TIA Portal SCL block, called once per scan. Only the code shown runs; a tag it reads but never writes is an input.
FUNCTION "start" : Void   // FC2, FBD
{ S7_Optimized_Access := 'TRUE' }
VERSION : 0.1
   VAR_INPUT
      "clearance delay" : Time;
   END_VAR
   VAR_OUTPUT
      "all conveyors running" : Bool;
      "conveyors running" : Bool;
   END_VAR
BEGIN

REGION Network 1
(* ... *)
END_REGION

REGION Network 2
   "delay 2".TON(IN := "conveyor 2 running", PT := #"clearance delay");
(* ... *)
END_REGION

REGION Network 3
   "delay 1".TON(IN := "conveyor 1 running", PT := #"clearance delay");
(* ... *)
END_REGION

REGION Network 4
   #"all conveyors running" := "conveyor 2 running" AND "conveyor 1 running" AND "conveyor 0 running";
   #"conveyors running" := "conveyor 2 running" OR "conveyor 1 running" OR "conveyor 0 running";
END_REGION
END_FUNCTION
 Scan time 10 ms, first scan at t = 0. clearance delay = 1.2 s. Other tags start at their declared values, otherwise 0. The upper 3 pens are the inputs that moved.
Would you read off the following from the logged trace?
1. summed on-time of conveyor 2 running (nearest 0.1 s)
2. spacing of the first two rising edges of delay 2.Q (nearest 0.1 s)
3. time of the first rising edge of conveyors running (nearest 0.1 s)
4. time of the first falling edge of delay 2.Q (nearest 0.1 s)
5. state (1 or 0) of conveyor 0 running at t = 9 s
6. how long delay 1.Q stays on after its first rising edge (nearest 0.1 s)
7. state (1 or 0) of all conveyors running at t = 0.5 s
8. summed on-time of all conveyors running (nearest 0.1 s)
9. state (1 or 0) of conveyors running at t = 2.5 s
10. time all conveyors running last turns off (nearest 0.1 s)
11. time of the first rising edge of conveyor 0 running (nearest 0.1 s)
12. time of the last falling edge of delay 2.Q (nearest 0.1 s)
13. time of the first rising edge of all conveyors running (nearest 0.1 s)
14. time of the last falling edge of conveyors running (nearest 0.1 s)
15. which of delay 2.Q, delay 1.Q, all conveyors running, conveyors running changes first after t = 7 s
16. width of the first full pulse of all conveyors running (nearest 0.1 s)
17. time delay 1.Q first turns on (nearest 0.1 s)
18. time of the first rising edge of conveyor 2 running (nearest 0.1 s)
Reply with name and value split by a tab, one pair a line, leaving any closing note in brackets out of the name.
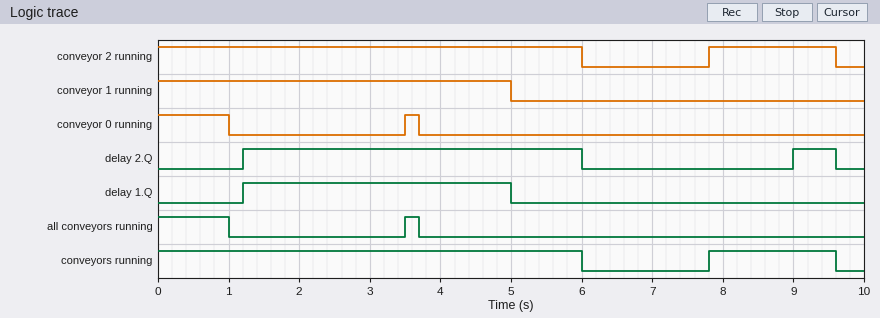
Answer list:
summed on-time of conveyor 2 running	7.8 s
spacing of the first two rising edges of delay 2.Q	7.8 s
time of the first rising edge of conveyors running	7.8 s
time of the first falling edge of delay 2.Q	6.0 s
state (1 or 0) of conveyor 0 running at t = 9 s	0
how long delay 1.Q stays on after its first rising edge	3.8 s
state (1 or 0) of all conveyors running at t = 0.5 s	1
summed on-time of all conveyors running	1.2 s
state (1 or 0) of conveyors running at t = 2.5 s	1
time all conveyors running last turns off	3.7 s
time of the first rising edge of conveyor 0 running	3.5 s
time of the last falling edge of delay 2.Q	9.6 s
time of the first rising edge of all conveyors running	3.5 s
time of the last falling edge of conveyors running	9.6 s
which of delay 2.Q, delay 1.Q, all conveyors running, conveyors running changes first after t = 7 s	conveyors running
width of the first full pulse of all conveyors running	0.2 s
time delay 1.Q first turns on	1.2 s
time of the first rising edge of conveyor 2 running	7.8 s
